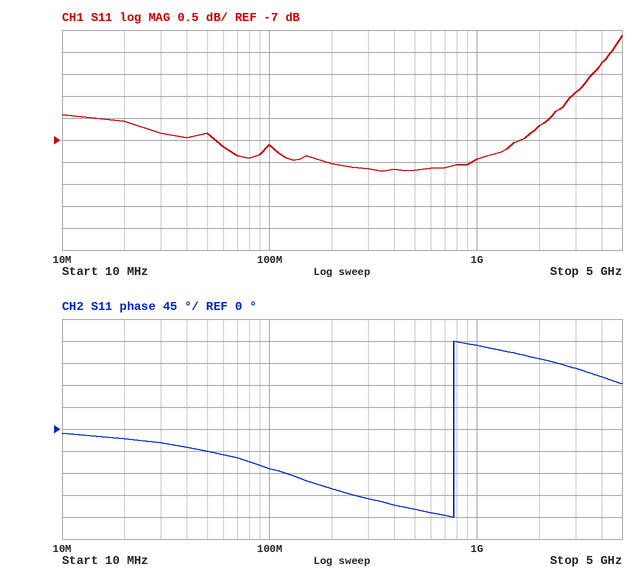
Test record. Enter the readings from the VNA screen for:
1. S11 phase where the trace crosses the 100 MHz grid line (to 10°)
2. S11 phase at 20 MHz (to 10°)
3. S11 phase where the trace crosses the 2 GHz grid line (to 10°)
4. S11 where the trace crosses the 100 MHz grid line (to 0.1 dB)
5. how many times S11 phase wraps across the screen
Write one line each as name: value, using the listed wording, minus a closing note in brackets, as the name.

S11 phase where the trace crosses the 100 MHz grid line: -80°
S11 phase at 20 MHz: -20°
S11 phase where the trace crosses the 2 GHz grid line: 140°
S11 where the trace crosses the 100 MHz grid line: -7.1 dB
how many times S11 phase wraps across the screen: 1
